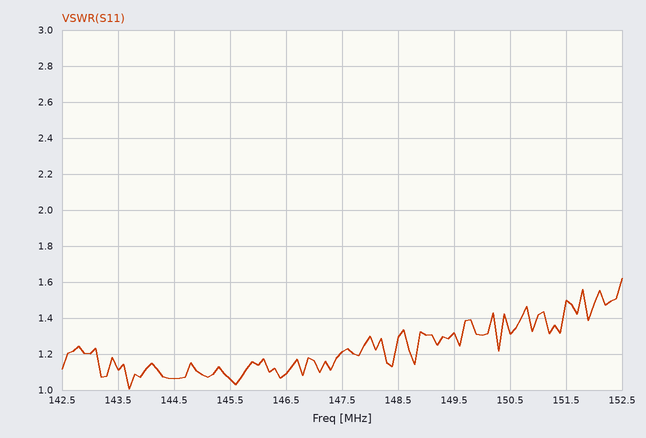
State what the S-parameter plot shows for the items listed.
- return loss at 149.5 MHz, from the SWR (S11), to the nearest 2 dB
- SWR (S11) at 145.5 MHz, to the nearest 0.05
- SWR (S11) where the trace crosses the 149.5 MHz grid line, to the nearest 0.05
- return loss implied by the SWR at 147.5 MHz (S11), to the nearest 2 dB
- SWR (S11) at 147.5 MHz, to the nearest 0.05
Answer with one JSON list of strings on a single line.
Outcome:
["18 dB", "1.05", "1.30", "20 dB", "1.20"]
